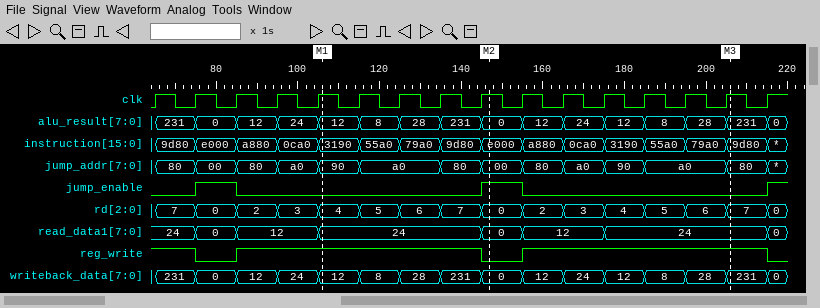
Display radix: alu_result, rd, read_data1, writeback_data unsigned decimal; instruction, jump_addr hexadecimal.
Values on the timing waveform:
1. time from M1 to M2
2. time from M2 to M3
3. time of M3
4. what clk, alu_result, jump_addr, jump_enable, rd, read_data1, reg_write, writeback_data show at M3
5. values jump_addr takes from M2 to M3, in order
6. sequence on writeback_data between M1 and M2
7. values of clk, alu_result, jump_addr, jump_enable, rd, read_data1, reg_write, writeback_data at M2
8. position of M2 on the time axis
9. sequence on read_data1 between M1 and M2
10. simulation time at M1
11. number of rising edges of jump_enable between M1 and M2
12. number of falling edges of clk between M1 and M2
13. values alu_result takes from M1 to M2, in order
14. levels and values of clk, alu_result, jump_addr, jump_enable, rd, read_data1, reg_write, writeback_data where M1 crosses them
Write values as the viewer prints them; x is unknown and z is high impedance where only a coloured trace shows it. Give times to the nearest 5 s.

40 s
60 s
205 s
clk=1, alu_result=231, jump_addr=80, jump_enable=0, rd=7, read_data1=24, reg_write=1, writeback_data=231
00, 80, a0, 90, a0, 80
12, 8, 28, 231, 0
clk=1, alu_result=0, jump_addr=00, jump_enable=1, rd=0, read_data1=0, reg_write=0, writeback_data=0
145 s
24, 0
105 s
1
4
12, 8, 28, 231, 0
clk=1, alu_result=12, jump_addr=90, jump_enable=0, rd=4, read_data1=24, reg_write=1, writeback_data=12
